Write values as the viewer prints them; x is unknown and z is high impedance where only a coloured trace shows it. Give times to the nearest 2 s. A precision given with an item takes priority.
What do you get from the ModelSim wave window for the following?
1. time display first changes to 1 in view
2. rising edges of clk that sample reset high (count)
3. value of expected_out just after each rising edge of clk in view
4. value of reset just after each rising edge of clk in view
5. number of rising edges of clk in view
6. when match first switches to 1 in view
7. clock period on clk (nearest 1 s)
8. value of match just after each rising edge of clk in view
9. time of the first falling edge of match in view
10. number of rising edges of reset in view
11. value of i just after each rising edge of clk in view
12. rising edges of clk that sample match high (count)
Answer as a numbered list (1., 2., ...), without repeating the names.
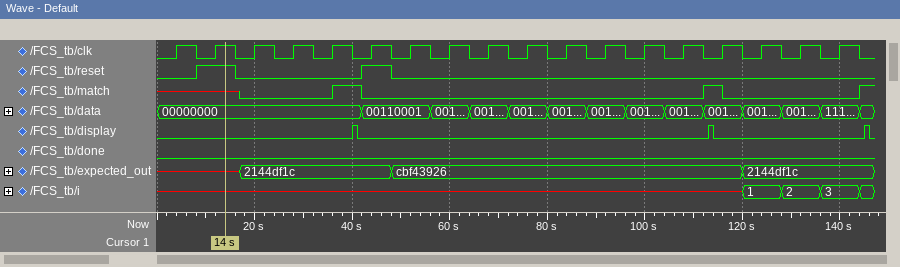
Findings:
1. 40 s
2. 2
3. x, x, 2144df1c, 2144df1c, 2144df1c, 2144df1c, cbf43926, cbf43926, cbf43926, cbf43926, cbf43926, cbf43926, cbf43926, cbf43926, cbf43926, 2144df1c, 2144df1c, 2144df1c
4. 0 1 0 0 0 1 0 0 0 0 0 0 0 0 0 0 0 0
5. 18
6. 36 s
7. 8 s
8. x x 0 0 1 0 0 0 0 0 0 0 0 0 0 0 0 0
9. 42 s
10. 2
11. x, x, x, x, x, x, x, x, x, x, x, x, x, x, x, 1, 2, 3
12. 1
